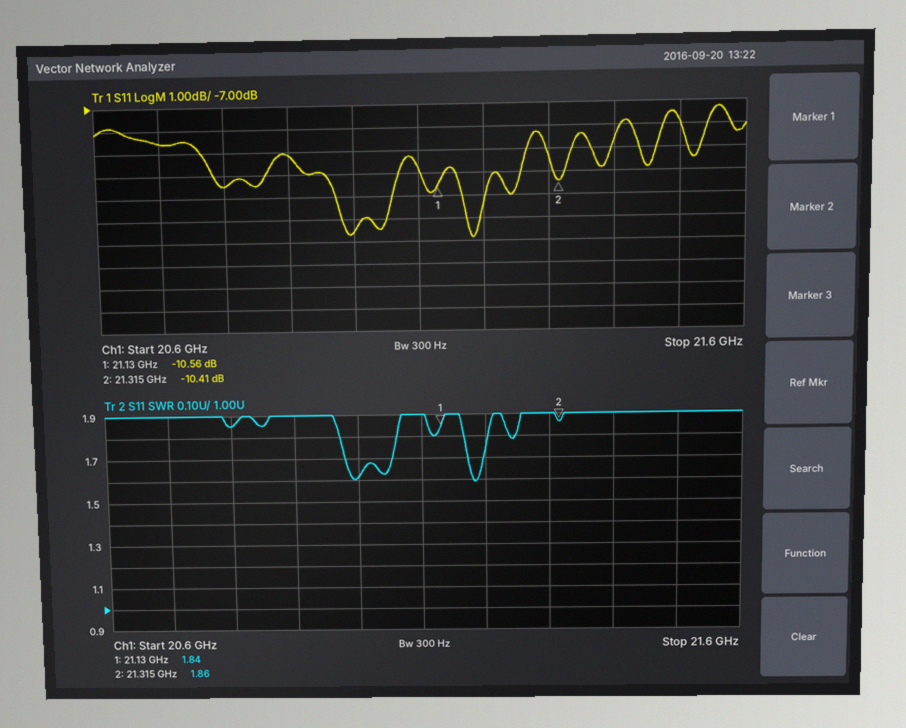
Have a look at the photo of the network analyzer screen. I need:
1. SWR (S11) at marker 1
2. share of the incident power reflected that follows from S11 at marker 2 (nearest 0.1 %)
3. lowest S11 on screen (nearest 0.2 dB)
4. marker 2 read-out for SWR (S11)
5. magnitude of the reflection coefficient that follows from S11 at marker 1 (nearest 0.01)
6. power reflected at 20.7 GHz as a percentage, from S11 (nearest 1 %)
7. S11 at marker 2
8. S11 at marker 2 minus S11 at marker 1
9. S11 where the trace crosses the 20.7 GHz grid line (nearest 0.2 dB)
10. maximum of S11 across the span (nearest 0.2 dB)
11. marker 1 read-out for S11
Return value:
1.84
9.1 %
-12.8 dB
1.86
0.30
14 %
-10.41 dB
0.15 dB
-8.6 dB
-7.2 dB
-10.56 dB
